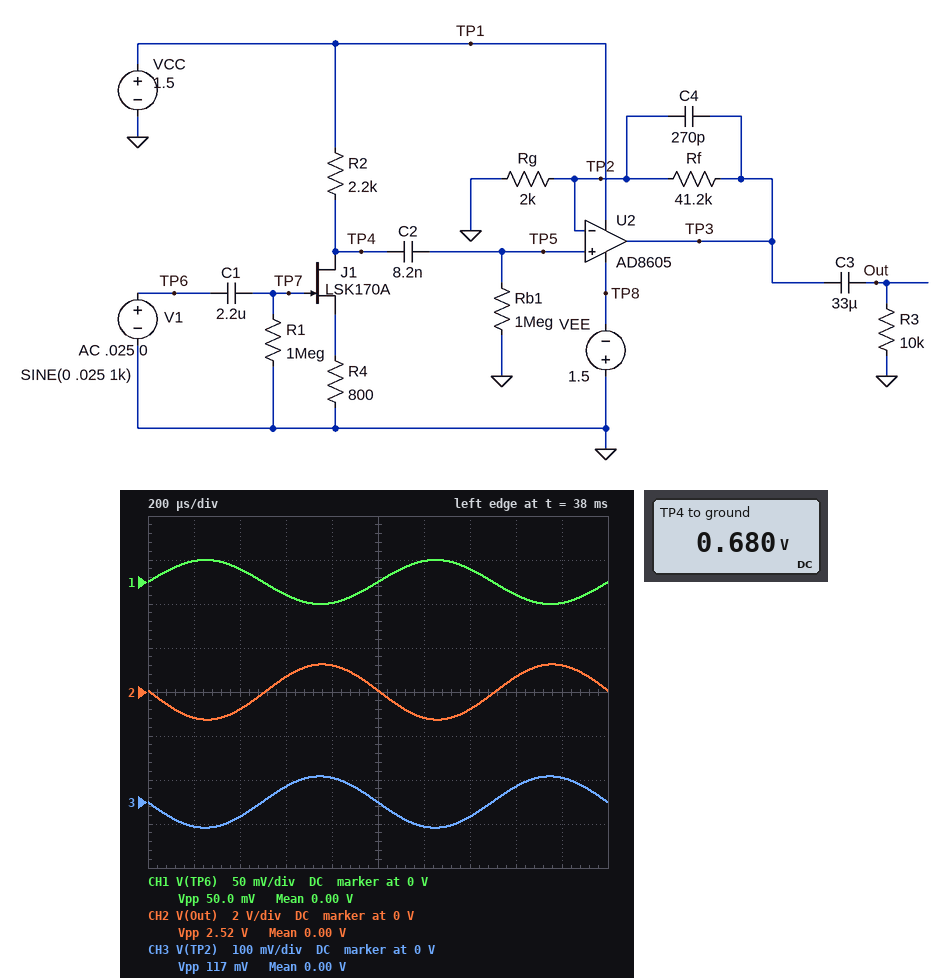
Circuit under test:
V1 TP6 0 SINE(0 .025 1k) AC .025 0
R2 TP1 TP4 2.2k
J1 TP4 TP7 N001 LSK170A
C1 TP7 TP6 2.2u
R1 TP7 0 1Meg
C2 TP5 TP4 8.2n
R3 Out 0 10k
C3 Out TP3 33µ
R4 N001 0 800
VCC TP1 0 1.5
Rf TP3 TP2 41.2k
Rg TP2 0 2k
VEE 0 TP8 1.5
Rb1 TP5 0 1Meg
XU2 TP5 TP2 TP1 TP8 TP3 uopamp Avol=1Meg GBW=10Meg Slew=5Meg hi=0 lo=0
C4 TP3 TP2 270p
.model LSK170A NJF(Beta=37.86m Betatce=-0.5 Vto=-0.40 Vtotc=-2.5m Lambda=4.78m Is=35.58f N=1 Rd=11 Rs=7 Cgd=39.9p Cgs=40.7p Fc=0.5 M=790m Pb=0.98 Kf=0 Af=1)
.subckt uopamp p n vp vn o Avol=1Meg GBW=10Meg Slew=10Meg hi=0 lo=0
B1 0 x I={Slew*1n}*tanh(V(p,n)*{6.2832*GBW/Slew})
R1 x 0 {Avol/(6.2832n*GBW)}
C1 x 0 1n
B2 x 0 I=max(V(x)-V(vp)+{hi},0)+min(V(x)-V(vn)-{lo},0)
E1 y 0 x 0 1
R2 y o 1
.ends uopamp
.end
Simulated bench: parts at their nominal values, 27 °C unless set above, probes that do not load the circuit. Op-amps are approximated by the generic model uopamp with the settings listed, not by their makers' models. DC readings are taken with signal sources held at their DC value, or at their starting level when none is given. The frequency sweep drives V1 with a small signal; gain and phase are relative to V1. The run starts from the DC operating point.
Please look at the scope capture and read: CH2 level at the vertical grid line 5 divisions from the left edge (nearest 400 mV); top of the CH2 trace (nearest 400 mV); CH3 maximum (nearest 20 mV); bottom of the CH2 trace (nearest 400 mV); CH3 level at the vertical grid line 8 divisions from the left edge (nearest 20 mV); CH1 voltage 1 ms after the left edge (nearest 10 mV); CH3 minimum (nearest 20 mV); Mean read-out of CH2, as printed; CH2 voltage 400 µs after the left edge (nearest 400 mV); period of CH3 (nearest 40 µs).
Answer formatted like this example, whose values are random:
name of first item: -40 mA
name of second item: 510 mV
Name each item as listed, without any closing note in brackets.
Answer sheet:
CH2 level at the vertical grid line 5 divisions from the left edge: 0 V
top of the CH2 trace: 1.2 V
CH3 maximum: 60 mV
bottom of the CH2 trace: -1.2 V
CH3 level at the vertical grid line 8 divisions from the left edge: 40 mV
CH1 voltage 1 ms after the left edge: 0 V
CH3 minimum: -60 mV
Mean read-out of CH2, as printed: 0.00 V
CH2 voltage 400 µs after the left edge: -800 mV
period of CH3: 1.00 ms
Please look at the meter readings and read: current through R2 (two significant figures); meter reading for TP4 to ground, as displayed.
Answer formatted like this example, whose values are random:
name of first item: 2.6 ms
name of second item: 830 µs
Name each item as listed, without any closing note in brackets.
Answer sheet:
current through R2: 370 µA
meter reading for TP4 to ground, as displayed: 0.680 V
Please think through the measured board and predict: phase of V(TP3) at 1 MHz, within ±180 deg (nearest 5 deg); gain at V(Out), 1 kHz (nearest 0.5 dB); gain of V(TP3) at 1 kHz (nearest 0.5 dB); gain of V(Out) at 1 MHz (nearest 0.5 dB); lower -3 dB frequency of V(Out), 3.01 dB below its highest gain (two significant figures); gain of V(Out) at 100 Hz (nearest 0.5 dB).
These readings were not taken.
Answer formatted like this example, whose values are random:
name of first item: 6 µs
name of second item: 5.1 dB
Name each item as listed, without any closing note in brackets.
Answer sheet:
phase of V(TP3) at 1 MHz, within ±180 deg: 125 deg
gain at V(Out), 1 kHz: 34.0 dB
gain of V(TP3) at 1 kHz: 34.0 dB
gain of V(Out) at 1 MHz: 7.0 dB
lower -3 dB frequency of V(Out), 3.01 dB below its highest gain: 19 Hz
gain of V(Out) at 100 Hz: 34.0 dB
